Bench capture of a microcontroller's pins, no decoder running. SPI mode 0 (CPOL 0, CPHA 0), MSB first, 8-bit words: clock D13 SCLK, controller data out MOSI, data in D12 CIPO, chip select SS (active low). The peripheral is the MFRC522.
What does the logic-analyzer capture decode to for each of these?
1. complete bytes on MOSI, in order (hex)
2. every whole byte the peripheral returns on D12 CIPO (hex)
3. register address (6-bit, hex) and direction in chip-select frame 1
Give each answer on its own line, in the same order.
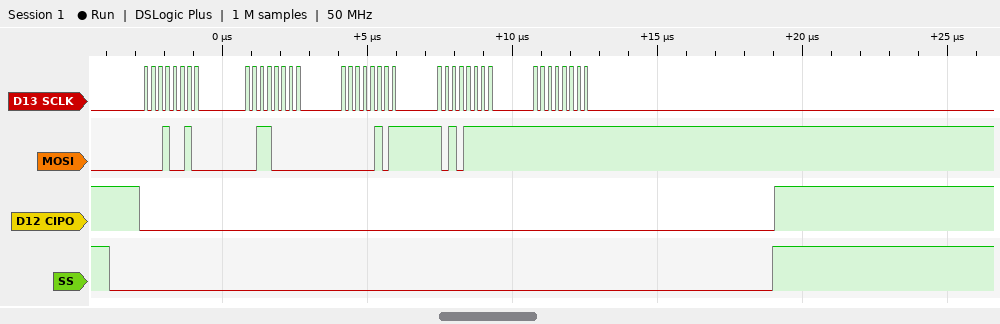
0x12 0x30 0x05 0xAF 0xFF
0x00 0x00 0x00 0x00 0x00
0x09 write
